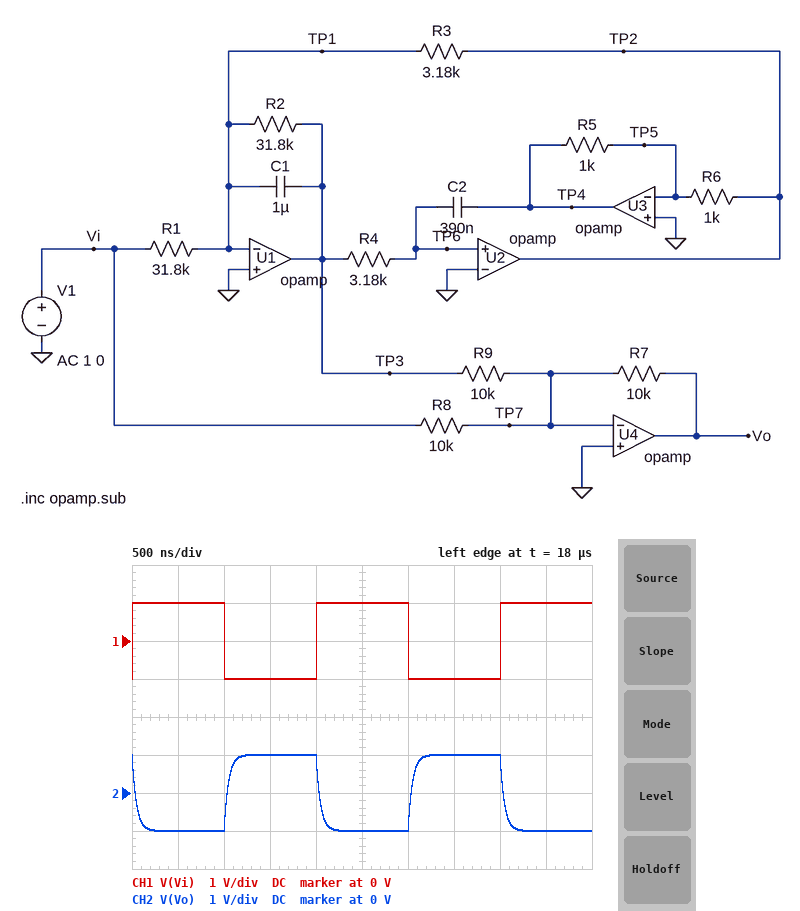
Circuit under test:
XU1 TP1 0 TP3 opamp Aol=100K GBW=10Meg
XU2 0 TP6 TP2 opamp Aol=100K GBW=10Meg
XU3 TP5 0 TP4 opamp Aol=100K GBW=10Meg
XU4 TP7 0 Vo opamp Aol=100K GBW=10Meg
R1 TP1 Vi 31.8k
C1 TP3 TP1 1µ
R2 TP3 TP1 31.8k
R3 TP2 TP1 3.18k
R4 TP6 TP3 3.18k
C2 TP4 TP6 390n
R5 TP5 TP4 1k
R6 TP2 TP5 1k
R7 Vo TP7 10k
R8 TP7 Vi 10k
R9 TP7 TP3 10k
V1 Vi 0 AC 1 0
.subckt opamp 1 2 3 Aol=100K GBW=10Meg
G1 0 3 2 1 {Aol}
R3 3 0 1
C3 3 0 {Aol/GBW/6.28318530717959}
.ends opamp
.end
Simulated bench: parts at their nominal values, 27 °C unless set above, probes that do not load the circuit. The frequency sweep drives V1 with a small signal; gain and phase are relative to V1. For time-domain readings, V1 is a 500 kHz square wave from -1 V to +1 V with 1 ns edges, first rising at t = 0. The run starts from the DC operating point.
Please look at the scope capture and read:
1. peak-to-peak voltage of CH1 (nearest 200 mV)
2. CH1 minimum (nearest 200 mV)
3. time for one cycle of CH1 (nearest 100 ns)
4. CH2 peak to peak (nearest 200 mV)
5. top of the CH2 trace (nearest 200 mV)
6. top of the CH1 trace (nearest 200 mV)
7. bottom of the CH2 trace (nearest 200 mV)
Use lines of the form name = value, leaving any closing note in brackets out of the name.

peak-to-peak voltage of CH1 = 2.0 V
CH1 minimum = -1.0 V
time for one cycle of CH1 = 2.0 µs
CH2 peak to peak = 2.0 V
top of the CH2 trace = 1.0 V
top of the CH1 trace = 1.0 V
bottom of the CH2 trace = -1.0 V
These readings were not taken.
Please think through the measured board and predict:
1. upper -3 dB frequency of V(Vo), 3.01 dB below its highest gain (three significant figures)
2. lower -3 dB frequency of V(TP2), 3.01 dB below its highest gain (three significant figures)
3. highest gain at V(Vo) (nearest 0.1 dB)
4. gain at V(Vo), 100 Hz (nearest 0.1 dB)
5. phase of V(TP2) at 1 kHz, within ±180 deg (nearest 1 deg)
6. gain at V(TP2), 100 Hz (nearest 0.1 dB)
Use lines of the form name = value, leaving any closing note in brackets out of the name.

upper -3 dB frequency of V(Vo), 3.01 dB below its highest gain = 3.33 MHz
lower -3 dB frequency of V(TP2), 3.01 dB below its highest gain = 77.5 Hz
highest gain at V(Vo) = 0 dB
gain at V(Vo), 100 Hz = -0.1 dB
phase of V(TP2) at 1 kHz, within ±180 deg = 0 deg
gain at V(TP2), 100 Hz = -15.0 dB
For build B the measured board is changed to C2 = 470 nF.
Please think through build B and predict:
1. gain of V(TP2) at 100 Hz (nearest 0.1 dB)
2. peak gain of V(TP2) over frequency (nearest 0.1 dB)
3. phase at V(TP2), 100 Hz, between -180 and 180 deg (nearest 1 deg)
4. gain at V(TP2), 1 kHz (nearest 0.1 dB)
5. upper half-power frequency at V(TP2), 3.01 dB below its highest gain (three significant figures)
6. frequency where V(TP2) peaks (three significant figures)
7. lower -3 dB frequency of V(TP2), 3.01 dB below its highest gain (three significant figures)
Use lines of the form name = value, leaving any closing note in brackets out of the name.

gain of V(TP2) at 100 Hz = -18.9 dB
peak gain of V(TP2) over frequency = 3.3 dB
phase at V(TP2), 100 Hz, between -180 and 180 deg = 6 deg
gain at V(TP2), 1 kHz = -65.4 dB
upper half-power frequency at V(TP2), 3.01 dB below its highest gain = 75.4 Hz
frequency where V(TP2) peaks = 72.9 Hz
lower -3 dB frequency of V(TP2), 3.01 dB below its highest gain = 70.4 Hz
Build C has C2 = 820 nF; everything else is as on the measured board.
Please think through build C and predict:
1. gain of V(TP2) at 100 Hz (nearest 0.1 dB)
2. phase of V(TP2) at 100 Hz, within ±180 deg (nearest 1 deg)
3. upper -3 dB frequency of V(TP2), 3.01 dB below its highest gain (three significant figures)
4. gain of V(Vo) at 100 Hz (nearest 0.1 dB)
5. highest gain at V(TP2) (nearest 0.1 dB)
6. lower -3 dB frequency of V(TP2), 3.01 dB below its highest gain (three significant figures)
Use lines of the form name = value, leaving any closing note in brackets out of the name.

gain of V(TP2) at 100 Hz = -27.2 dB
phase of V(TP2) at 100 Hz, within ±180 deg = 4 deg
upper -3 dB frequency of V(TP2), 3.01 dB below its highest gain = 57.6 Hz
gain of V(Vo) at 100 Hz = 0 dB
highest gain at V(TP2) = 0.9 dB
lower -3 dB frequency of V(TP2), 3.01 dB below its highest gain = 52.6 Hz
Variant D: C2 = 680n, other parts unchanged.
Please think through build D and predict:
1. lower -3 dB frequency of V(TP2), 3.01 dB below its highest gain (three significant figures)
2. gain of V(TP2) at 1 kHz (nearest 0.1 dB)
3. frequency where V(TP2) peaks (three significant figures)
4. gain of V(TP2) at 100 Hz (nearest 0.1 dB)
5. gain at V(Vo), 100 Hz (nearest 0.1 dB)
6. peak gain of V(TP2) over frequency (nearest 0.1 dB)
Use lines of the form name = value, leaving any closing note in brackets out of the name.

lower -3 dB frequency of V(TP2), 3.01 dB below its highest gain = 58.0 Hz
gain of V(TP2) at 1 kHz = -68.6 dB
frequency where V(TP2) peaks = 60.6 Hz
gain of V(TP2) at 100 Hz = -24.7 dB
gain at V(Vo), 100 Hz = 0 dB
peak gain of V(TP2) over frequency = 1.7 dB
